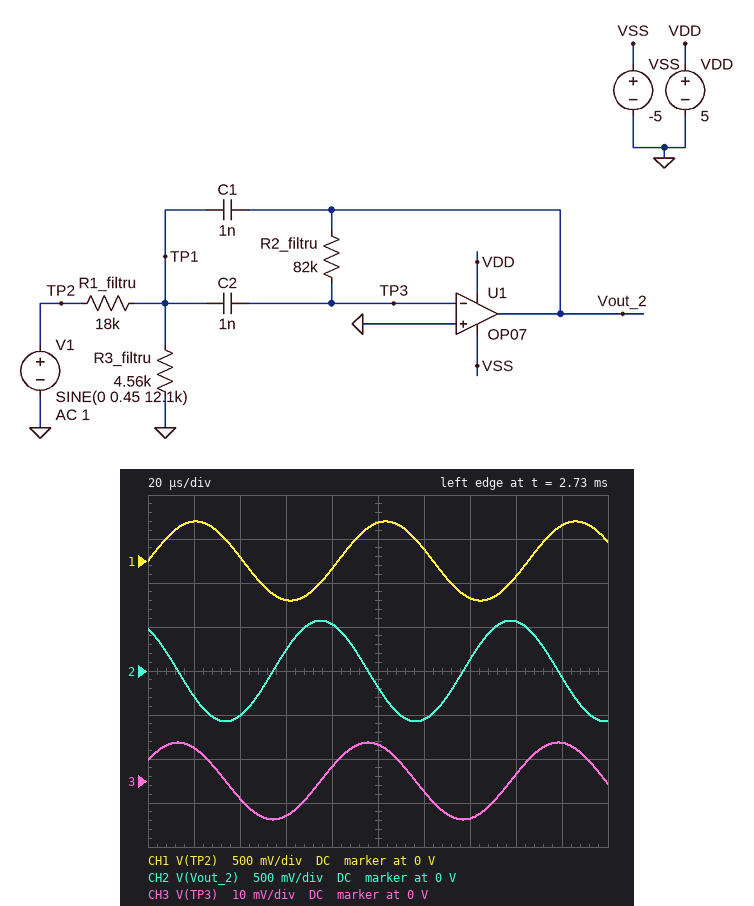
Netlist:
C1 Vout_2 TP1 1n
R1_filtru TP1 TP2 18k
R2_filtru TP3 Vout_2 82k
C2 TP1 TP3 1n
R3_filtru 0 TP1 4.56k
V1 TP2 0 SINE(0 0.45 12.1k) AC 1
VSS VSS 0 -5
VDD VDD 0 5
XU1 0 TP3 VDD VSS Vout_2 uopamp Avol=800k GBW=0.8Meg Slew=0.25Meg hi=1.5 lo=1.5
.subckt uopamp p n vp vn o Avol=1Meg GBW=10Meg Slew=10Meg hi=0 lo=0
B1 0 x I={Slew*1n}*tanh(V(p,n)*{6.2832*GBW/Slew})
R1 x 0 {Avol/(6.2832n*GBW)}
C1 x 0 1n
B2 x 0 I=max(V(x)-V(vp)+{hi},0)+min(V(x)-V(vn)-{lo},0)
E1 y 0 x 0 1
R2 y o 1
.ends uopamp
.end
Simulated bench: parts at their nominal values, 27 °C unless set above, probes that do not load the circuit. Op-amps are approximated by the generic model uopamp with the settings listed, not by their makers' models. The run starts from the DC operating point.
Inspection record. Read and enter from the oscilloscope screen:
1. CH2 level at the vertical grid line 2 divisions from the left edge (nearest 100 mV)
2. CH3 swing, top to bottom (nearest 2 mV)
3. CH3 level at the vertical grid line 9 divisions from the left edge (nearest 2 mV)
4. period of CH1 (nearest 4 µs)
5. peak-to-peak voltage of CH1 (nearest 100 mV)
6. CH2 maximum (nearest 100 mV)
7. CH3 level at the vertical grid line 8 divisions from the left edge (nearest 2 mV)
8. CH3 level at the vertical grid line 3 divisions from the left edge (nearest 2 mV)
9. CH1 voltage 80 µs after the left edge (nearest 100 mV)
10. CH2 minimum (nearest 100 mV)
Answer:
-500 mV
18 mV
8 mV
84 µs
900 mV
600 mV
2 mV
-8 mV
-100 mV
-600 mV
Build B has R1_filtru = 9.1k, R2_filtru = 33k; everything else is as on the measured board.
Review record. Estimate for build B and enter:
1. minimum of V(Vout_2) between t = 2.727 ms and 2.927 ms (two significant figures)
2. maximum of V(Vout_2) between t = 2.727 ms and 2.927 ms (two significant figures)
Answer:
-630 mV
630 mV
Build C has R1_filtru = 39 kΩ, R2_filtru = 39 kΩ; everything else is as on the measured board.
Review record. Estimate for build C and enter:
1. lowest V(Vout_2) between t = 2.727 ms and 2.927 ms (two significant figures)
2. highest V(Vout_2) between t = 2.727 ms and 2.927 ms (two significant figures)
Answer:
-220 mV
220 mV
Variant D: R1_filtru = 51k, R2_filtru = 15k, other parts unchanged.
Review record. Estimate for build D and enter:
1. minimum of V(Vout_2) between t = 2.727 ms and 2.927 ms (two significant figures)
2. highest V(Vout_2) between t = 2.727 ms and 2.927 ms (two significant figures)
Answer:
-47 mV
47 mV
